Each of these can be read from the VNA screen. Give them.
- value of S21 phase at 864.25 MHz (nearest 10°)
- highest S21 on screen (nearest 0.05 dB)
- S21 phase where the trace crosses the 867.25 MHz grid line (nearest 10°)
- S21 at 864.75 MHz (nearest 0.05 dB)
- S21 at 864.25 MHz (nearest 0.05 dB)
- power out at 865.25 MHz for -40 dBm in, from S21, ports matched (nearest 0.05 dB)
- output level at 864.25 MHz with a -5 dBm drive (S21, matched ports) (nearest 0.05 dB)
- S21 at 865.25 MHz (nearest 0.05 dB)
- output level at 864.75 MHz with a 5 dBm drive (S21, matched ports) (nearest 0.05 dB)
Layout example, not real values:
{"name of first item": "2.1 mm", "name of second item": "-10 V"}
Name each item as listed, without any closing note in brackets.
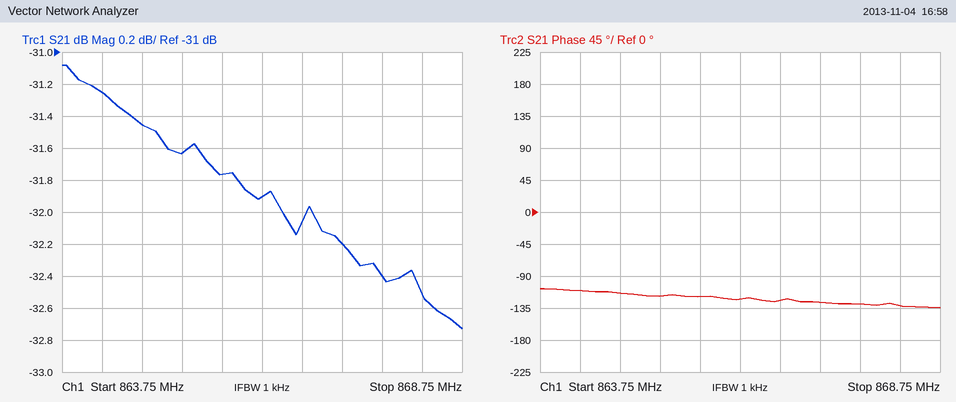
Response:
{"value of S21 phase at 864.25 MHz": "-110°", "highest S21 on screen": "-31.10 dB", "S21 phase where the trace crosses the 867.25 MHz grid line": "-130°", "S21 at 864.75 MHz": "-31.45 dB", "S21 at 864.25 MHz": "-31.25 dB", "power out at 865.25 MHz for -40 dBm in, from S21, ports matched": "-71.65 dBm", "output level at 864.25 MHz with a -5 dBm drive (S21, matched ports)": "-36.25 dBm", "S21 at 865.25 MHz": "-31.65 dB", "output level at 864.75 MHz with a 5 dBm drive (S21, matched ports)": "-26.45 dBm"}
